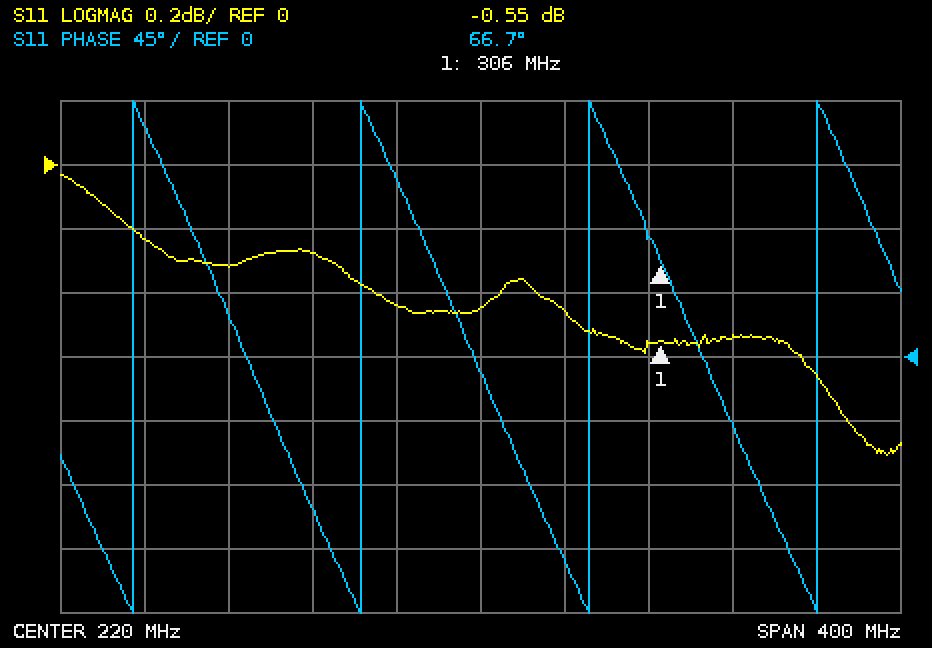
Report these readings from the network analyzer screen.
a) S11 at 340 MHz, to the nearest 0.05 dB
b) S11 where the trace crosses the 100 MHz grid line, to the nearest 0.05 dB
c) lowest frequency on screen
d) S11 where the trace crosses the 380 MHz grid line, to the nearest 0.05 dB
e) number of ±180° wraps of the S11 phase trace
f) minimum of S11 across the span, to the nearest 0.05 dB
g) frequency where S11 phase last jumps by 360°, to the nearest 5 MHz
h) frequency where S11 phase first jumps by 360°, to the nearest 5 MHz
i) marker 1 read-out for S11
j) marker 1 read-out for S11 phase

-0.55 dB
-0.30 dB
20 MHz
-0.65 dB
4
-0.90 dB
380 MHz
55 MHz
-0.55 dB
66.7°
